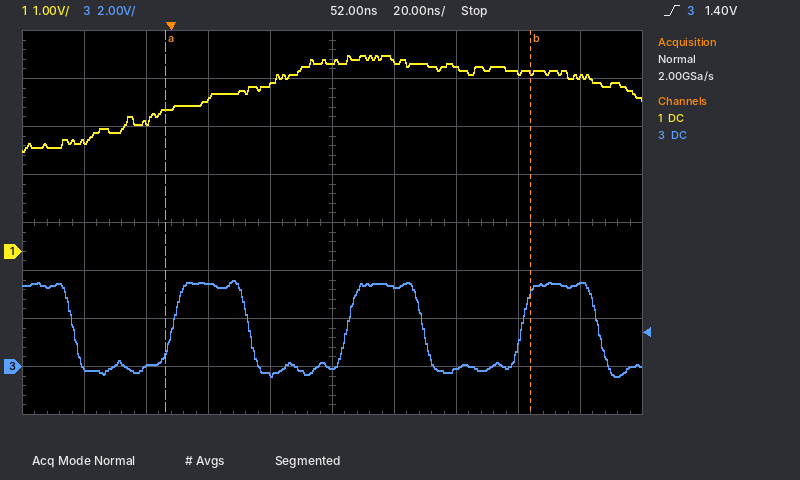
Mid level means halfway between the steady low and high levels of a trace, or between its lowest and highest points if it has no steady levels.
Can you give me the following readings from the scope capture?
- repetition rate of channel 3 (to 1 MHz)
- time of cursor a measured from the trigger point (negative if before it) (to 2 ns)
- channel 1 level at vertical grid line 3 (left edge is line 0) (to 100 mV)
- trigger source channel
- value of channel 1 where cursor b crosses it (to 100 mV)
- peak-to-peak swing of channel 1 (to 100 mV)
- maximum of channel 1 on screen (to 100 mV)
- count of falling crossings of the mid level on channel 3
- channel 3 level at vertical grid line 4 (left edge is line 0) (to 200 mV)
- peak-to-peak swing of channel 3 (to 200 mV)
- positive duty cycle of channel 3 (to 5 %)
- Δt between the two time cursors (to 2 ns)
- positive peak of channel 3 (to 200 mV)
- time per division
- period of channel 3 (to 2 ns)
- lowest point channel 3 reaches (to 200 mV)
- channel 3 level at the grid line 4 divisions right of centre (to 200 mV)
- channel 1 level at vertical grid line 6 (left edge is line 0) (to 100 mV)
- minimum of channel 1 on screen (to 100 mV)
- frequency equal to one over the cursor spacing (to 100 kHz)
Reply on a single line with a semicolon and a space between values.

18 MHz; -2 ns; 3.2 V; channel 3; 3.7 V; 2.0 V; 4.1 V; 4; -400 mV; 4.0 V; 45 %; 118 ns; 3.6 V; 20 ns; 56 ns; -400 mV; 3.4 V; 4.0 V; 2.1 V; 8.5 MHz
